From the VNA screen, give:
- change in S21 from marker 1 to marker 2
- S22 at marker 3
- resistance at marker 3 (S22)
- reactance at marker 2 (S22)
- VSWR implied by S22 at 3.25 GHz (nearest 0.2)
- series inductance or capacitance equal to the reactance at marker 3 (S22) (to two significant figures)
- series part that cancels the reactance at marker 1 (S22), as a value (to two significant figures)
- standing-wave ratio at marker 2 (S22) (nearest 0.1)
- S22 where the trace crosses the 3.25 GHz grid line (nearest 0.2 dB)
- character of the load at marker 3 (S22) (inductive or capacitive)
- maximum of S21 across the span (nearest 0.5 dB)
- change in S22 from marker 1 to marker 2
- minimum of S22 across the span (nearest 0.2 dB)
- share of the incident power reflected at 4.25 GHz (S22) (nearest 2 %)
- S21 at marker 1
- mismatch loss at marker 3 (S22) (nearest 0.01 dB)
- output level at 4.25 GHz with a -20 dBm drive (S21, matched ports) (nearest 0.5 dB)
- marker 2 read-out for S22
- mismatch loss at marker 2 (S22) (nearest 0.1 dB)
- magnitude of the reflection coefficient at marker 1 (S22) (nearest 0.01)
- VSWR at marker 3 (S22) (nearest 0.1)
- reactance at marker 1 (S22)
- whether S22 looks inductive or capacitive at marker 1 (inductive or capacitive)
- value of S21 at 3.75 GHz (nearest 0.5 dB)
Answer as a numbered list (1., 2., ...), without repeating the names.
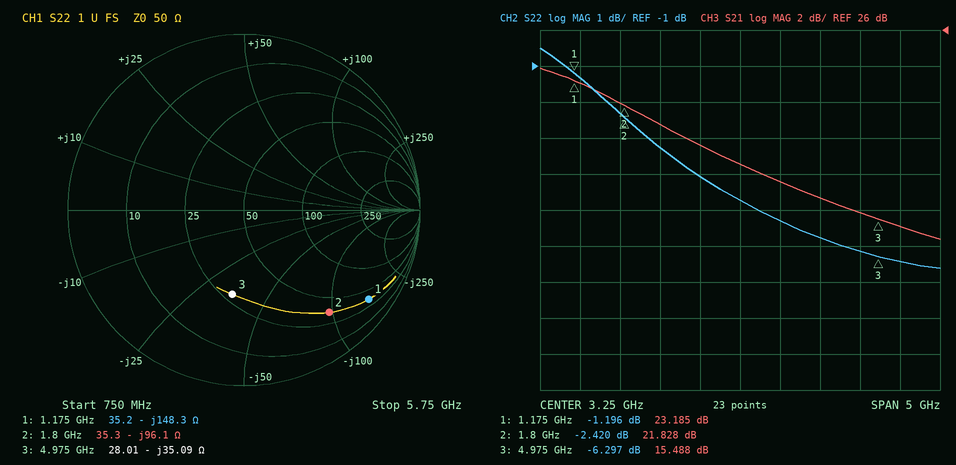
1. -1.357 dB
2. -6.297 dB
3. 28.01 Ω
4. -96.1 Ω
5. 3.8
6. 910 fF
7. 20 nH
8. 7.2
9. -4.8 dB
10. capacitive
11. 24.0 dB
12. -1.224 dB
13. -6.6 dB
14. 26 %
15. 23.185 dB
16. 1.16 dB
17. -3.5 dBm
18. -2.420 dB
19. 3.7 dB
20. 0.87
21. 2.9
22. -148.3 Ω
23. capacitive
24. 17.5 dB
